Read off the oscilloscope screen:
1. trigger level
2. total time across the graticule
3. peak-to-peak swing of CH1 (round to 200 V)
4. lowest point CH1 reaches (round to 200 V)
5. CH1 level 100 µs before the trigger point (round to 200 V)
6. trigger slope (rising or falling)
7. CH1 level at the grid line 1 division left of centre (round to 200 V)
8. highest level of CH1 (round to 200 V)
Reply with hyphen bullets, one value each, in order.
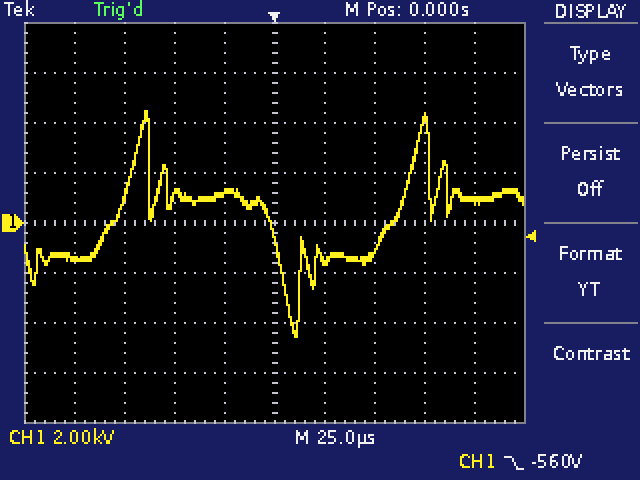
- -560 V
- 250 µs
- 9.0 kV
- -4.6 kV
- -1.4 kV
- falling
- 1.2 kV
- 4.4 kV
